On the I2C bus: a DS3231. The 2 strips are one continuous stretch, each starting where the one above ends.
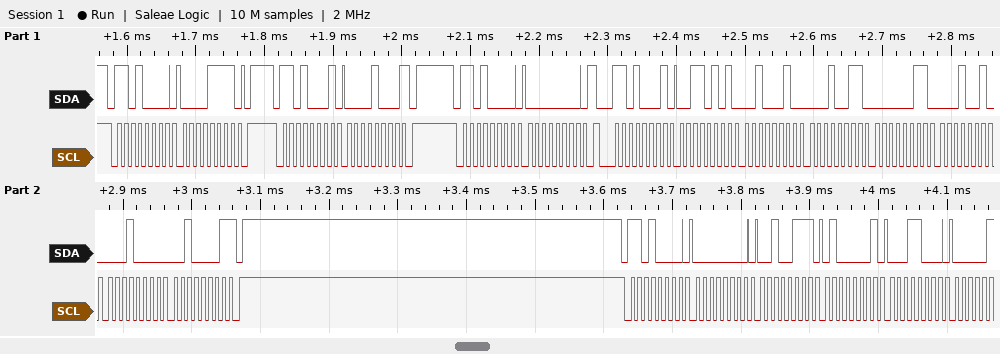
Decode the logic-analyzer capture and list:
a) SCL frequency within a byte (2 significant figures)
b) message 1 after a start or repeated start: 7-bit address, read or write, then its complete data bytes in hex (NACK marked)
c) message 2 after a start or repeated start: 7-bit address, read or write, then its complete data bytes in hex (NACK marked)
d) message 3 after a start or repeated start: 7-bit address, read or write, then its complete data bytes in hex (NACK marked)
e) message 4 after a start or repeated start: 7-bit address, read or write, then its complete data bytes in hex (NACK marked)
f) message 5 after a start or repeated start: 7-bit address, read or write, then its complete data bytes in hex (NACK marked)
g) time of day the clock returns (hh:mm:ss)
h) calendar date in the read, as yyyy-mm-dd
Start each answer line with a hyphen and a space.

- 100 kHz
- 0x68 write: 0F
- 0x68 read: 08 NACK
- 0x68 write: 00
- 0x68 read: 35 22 13 03 12 10 21 NACK
- 0x68 write: 00 27 41 18
- 13:22:35
- 2021-10-12
